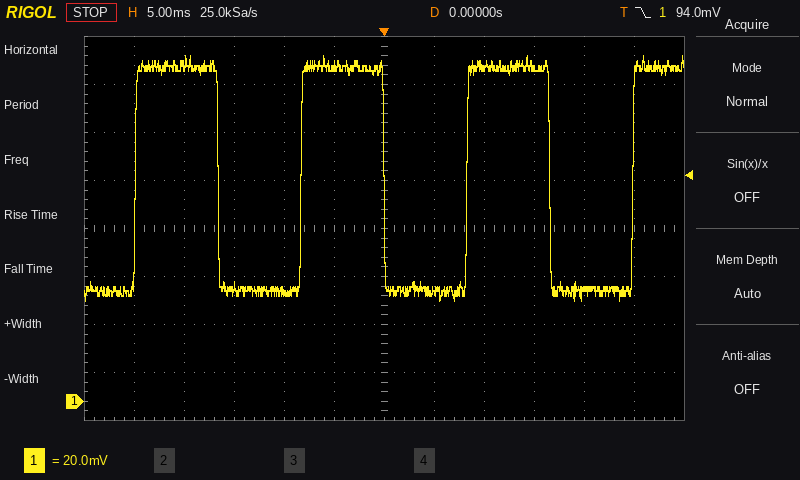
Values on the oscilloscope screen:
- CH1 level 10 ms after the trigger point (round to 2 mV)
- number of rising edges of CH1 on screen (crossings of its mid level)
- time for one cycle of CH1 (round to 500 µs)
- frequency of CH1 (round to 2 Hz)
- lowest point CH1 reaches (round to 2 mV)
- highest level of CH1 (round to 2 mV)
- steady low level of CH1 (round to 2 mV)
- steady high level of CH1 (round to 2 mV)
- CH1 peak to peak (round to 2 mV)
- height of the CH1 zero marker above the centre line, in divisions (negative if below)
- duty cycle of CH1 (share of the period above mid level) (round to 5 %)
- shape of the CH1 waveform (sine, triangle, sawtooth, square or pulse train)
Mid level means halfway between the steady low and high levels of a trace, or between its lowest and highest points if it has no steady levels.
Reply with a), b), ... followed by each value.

a) 140 mV
b) 4
c) 16.5 ms
d) 60 Hz
e) 42 mV
f) 144 mV
g) 46 mV
h) 140 mV
i) 102 mV
j) -3.6 div
k) 50 %
l) square
